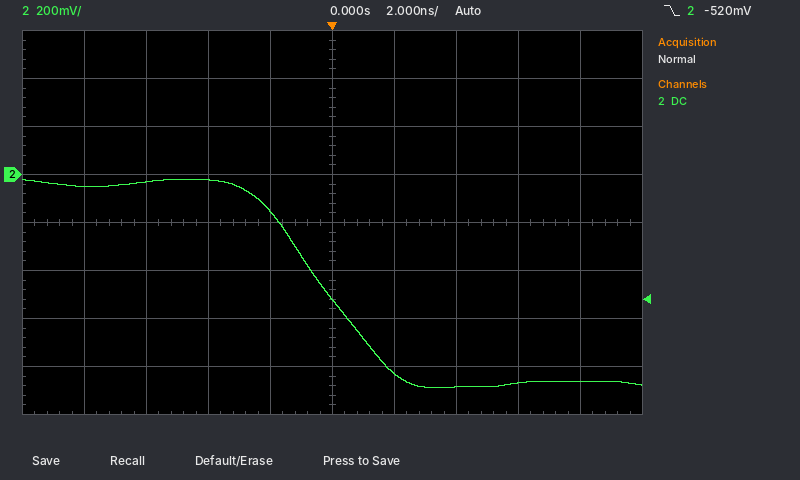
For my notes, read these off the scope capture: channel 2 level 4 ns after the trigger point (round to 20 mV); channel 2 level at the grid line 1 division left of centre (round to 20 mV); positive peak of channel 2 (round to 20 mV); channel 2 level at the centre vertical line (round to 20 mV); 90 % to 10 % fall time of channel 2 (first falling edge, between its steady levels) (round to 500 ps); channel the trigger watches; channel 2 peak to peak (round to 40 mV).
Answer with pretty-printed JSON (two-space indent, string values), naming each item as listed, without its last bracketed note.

{
  "channel 2 level 4 ns after the trigger point": "-880 mV",
  "channel 2 level at the grid line 1 division left of centre": "-160 mV",
  "positive peak of channel 2": "-20 mV",
  "channel 2 level at the centre vertical line": "-520 mV",
  "90 % to 10 % fall time of channel 2 (first falling edge, between its steady levels)": "4.0 ns",
  "channel the trigger watches": "channel 2",
  "channel 2 peak to peak": "880 mV"
}
